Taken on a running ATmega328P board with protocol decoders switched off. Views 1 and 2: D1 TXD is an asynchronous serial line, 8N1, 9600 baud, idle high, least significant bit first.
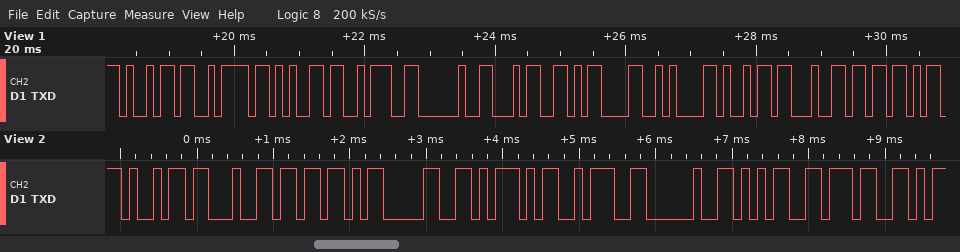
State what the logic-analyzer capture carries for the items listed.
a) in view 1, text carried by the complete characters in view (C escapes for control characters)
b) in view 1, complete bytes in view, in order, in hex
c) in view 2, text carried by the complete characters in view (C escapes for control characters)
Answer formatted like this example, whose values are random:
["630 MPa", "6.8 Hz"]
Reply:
["\"ize: 4\\r\\nid[\"", "69 7A 65 3A 20 34 0D 0A 69 64 5B", "\"id[0]: 57\""]
